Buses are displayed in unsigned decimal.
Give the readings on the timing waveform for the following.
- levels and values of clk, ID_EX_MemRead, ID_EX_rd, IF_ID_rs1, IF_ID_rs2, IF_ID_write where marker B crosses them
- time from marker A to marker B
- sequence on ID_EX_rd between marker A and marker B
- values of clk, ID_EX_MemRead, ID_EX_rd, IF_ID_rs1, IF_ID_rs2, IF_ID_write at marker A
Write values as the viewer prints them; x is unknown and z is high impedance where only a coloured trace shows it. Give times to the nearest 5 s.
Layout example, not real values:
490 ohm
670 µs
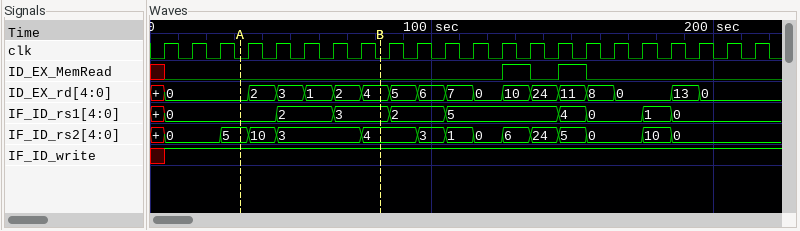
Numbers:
clk=0, ID_EX_MemRead=0, ID_EX_rd=4, IF_ID_rs1=3, IF_ID_rs2=4, IF_ID_write=1
50 s
0, 2, 3, 1, 2, 4
clk=0, ID_EX_MemRead=0, ID_EX_rd=0, IF_ID_rs1=0, IF_ID_rs2=5, IF_ID_write=1
